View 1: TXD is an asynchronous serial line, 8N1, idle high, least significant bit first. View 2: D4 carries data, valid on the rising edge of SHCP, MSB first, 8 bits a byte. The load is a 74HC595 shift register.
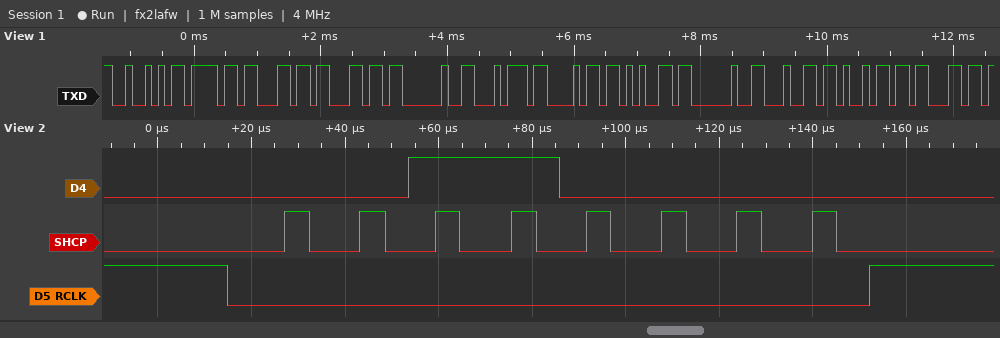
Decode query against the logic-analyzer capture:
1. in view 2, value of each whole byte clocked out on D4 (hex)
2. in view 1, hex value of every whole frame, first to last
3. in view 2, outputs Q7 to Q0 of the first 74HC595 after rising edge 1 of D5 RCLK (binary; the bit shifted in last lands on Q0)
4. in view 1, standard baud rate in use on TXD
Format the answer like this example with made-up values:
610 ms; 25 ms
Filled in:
0x30; 52 6F 6C 6C 20 74 68 65 20 64 69 63; 00110000; 9600 baud
